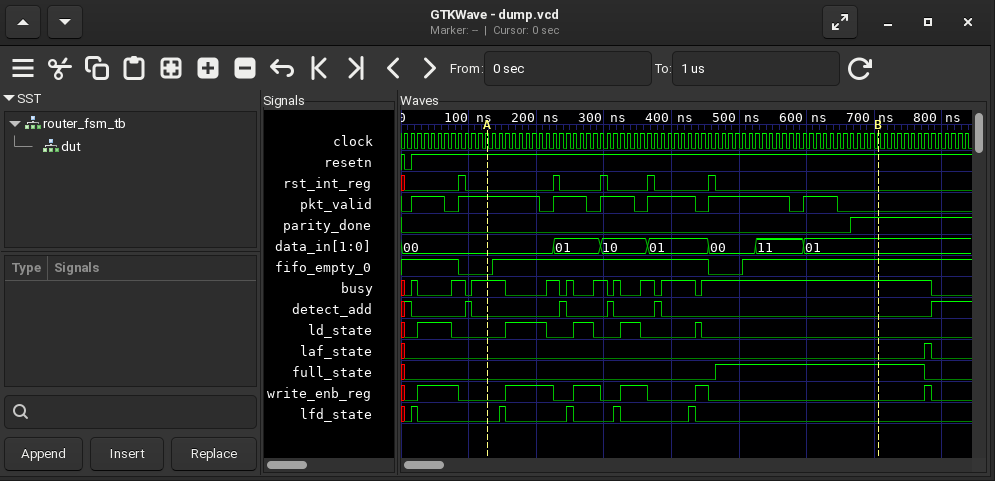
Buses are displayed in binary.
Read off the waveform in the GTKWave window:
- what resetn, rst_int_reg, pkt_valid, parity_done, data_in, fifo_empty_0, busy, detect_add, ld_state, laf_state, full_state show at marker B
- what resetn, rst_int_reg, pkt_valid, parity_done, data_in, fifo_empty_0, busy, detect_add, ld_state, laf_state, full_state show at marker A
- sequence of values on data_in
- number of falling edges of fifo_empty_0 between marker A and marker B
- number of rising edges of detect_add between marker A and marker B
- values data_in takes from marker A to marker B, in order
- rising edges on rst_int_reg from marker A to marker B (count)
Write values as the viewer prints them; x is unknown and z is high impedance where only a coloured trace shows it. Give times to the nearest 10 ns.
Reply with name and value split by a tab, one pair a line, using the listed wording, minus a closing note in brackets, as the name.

what resetn, rst_int_reg, pkt_valid, parity_done, data_in, fifo_empty_0, busy, detect_add, ld_state, laf_state, full_state show at marker B	resetn=1, rst_int_reg=0, pkt_valid=0, parity_done=1, data_in=01, fifo_empty_0=1, busy=1, detect_add=0, ld_state=0, laf_state=0, full_state=1
what resetn, rst_int_reg, pkt_valid, parity_done, data_in, fifo_empty_0, busy, detect_add, ld_state, laf_state, full_state show at marker A	resetn=1, rst_int_reg=0, pkt_valid=1, parity_done=0, data_in=00, fifo_empty_0=0, busy=1, detect_add=0, ld_state=0, laf_state=0, full_state=0
sequence of values on data_in	00, 01, 10, 01, 00, 11, 01
number of falling edges of fifo_empty_0 between marker A and marker B	1
number of rising edges of detect_add between marker A and marker B	3
values data_in takes from marker A to marker B, in order	00, 01, 10, 01, 00, 11, 01
rising edges on rst_int_reg from marker A to marker B	4
